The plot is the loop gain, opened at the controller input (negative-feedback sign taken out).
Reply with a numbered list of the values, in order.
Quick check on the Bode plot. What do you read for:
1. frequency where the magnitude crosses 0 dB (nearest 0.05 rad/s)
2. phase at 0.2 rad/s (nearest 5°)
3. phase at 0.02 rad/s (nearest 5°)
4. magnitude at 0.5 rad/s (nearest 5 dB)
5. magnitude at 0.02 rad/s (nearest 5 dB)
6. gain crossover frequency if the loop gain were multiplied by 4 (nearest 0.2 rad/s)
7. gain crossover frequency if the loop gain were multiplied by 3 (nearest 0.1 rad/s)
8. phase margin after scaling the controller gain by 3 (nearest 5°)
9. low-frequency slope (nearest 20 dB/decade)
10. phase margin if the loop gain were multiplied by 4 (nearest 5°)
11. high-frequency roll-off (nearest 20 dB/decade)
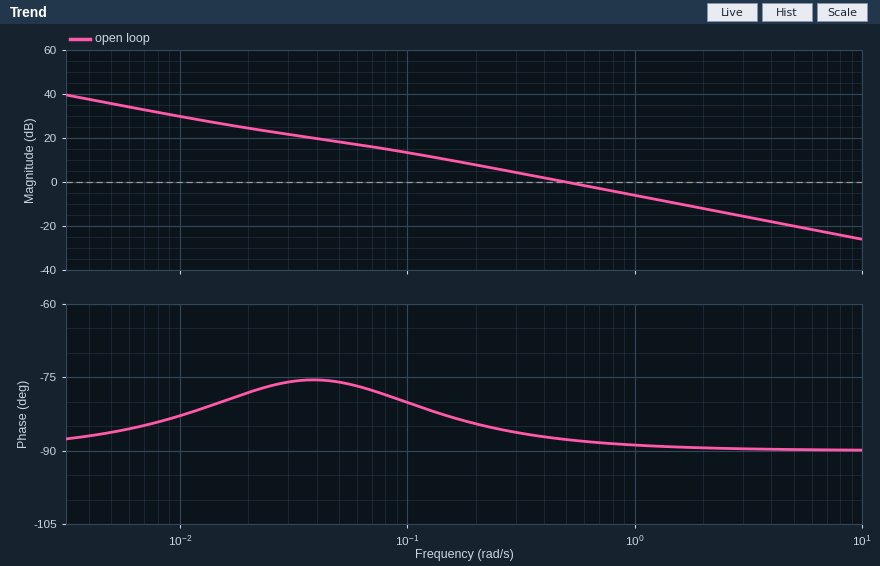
1. 0.50 rad/s
2. -85°
3. -80°
4. 0 dB
5. 25 dB
6. 2.0 rad/s
7. 1.5 rad/s
8. 90°
9. -20 dB/decade
10. 90°
11. -20 dB/decade
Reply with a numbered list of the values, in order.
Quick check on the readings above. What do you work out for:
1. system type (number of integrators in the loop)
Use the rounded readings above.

1. 1
